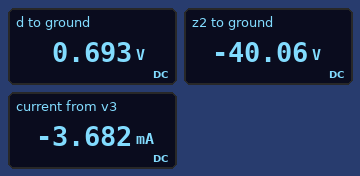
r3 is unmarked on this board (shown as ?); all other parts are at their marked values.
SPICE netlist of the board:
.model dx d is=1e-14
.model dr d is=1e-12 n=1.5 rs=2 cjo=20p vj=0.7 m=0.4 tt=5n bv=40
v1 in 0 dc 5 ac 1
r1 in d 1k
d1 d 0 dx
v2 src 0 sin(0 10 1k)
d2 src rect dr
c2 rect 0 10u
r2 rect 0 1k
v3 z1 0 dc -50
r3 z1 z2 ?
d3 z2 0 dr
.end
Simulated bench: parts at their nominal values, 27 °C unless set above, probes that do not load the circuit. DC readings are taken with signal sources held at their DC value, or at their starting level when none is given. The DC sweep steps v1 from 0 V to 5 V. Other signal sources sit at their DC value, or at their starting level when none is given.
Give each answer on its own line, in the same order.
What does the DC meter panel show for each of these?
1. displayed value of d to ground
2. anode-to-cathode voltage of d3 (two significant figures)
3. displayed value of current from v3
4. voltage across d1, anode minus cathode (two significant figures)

0.693 V
-40 V
-3.682 mA
690 mV
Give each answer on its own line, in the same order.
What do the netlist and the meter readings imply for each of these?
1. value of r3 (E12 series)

2.7 kΩ
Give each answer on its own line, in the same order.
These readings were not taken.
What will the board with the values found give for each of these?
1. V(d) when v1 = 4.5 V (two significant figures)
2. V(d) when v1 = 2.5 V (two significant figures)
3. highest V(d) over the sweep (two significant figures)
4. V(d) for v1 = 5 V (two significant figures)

690 mV
670 mV
690 mV
690 mV
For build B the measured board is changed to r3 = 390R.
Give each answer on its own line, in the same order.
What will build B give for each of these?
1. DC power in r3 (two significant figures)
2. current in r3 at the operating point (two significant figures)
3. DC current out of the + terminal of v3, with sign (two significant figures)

250 mW
25 mA
-25 mA
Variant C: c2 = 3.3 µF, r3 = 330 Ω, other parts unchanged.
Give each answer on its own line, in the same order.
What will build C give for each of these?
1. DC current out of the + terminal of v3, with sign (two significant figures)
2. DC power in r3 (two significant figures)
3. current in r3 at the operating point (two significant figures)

-30 mA
290 mW
30 mA
